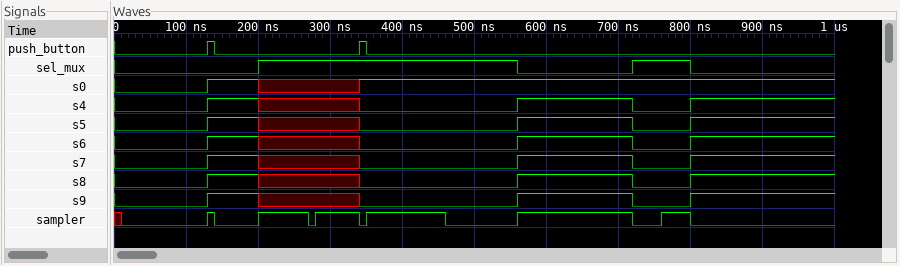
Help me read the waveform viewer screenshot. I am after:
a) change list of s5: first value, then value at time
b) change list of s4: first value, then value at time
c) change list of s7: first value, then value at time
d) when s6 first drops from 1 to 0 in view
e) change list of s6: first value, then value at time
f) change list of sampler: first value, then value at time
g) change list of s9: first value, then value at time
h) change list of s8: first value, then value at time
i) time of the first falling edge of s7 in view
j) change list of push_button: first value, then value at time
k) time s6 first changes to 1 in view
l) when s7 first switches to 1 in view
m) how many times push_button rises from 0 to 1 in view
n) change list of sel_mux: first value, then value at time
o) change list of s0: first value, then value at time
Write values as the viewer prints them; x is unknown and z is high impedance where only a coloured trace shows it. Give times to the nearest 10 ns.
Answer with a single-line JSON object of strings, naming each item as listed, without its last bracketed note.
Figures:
{"change list of s5: first value, then value at time": "0, 1 at 130 ns, x at 200 ns, 0 at 340 ns, 1 at 560 ns, 0 at 720 ns, 1 at 800 ns", "change list of s4: first value, then value at time": "0, 1 at 130 ns, x at 200 ns, 0 at 340 ns, 1 at 560 ns, 0 at 720 ns, 1 at 800 ns", "change list of s7: first value, then value at time": "0, 1 at 130 ns, x at 200 ns, 0 at 340 ns, 1 at 560 ns, 0 at 720 ns, 1 at 800 ns", "when s6 first drops from 1 to 0 in view": "720 ns", "change list of s6: first value, then value at time": "0, 1 at 130 ns, x at 200 ns, 0 at 340 ns, 1 at 560 ns, 0 at 720 ns, 1 at 800 ns", "change list of sampler: first value, then value at time": "x, 0 at 10 ns, 1 at 130 ns, 0 at 140 ns, 1 at 200 ns, 0 at 270 ns, 1 at 280 ns, 0 at 340 ns, 1 at 350 ns, 0 at 460 ns, 1 at 560 ns, 0 at 720 ns, 1 at 760 ns, 0 at 800 ns", "change list of s9: first value, then value at time": "0, 1 at 130 ns, x at 200 ns, 0 at 340 ns, 1 at 560 ns, 0 at 720 ns, 1 at 800 ns", "change list of s8: first value, then value at time": "0, 1 at 130 ns, x at 200 ns, 0 at 340 ns, 1 at 560 ns, 0 at 720 ns, 1 at 800 ns", "time of the first falling edge of s7 in view": "720 ns", "change list of push_button: first value, then value at time": "0, 1 at 130 ns, 0 at 140 ns, 1 at 340 ns, 0 at 350 ns", "time s6 first changes to 1 in view": "130 ns", "when s7 first switches to 1 in view": "130 ns", "how many times push_button rises from 0 to 1 in view": "2", "change list of sel_mux: first value, then value at time": "0, 1 at 200 ns, 0 at 560 ns, 1 at 720 ns, 0 at 800 ns", "change list of s0: first value, then value at time": "0, 1 at 130 ns, x at 200 ns, 1 at 340 ns"}
